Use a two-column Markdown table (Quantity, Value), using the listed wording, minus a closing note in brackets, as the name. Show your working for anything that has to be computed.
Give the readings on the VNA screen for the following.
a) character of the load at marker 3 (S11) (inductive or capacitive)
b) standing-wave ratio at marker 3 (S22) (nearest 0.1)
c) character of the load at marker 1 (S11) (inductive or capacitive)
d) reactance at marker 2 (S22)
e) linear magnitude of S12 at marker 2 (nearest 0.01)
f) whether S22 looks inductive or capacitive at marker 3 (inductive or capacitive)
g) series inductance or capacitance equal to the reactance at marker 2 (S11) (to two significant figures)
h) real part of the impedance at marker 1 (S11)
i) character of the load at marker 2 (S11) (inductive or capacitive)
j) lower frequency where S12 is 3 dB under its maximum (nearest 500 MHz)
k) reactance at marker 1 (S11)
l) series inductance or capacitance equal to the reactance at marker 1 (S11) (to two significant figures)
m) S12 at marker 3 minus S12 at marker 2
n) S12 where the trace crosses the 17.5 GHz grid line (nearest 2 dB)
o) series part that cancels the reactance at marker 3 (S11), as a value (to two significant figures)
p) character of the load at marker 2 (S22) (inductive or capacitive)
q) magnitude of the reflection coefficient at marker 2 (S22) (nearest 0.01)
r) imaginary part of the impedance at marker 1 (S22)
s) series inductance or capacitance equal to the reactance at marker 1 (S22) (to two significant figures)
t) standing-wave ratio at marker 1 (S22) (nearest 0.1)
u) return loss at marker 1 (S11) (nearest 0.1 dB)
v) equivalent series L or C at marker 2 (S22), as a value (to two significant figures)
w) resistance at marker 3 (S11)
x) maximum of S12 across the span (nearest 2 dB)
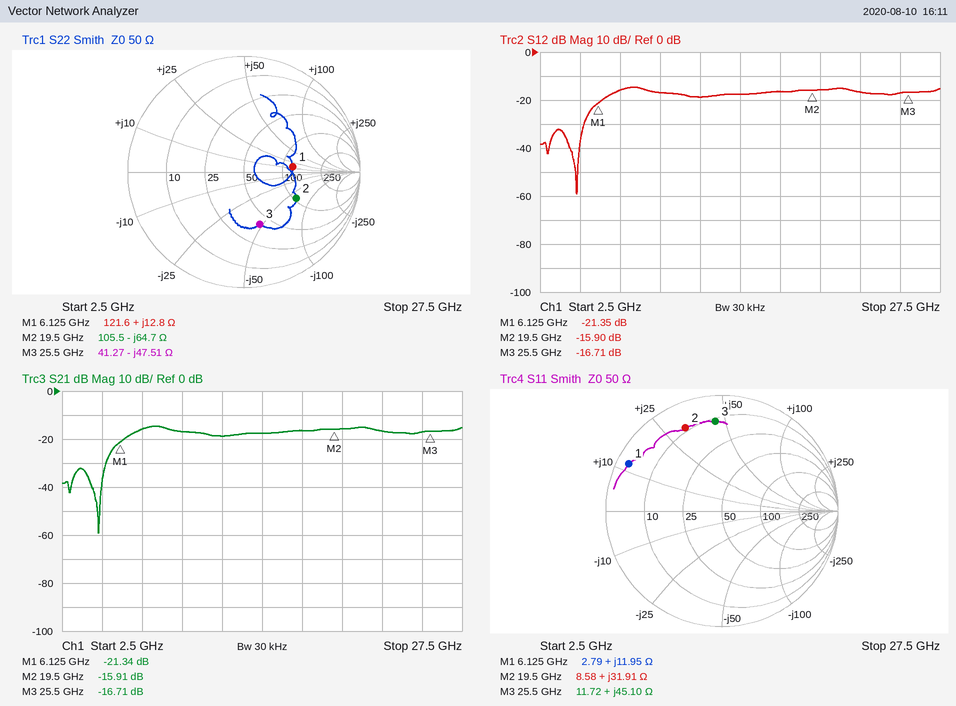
| Quantity | Value |
|---|---|
| character of the load at marker 3 (S11) | inductive |
| standing-wave ratio at marker 3 (S22) | 2.8 |
| character of the load at marker 1 (S11) | inductive |
| reactance at marker 2 | -64.7 Ω |
| linear magnitude of S12 at marker 2 | 10^(-15.9/20) ≈ 0.16 |
| whether S22 looks inductive or capacitive at marker 3 | capacitive |
| series inductance or capacitance equal to the reactance at marker 2 (S11) | L = 31.91 Ω/(2π × 19.5 GHz) ≈ 260 pH |
| real part of the impedance at marker 1 | 2.79 Ω |
| character of the load at marker 2 (S11) | inductive |
| lower frequency where S12 is 3 dB under its maximum | 7.0 GHz |
| reactance at marker 1 | +11.95 Ω |
| series inductance or capacitance equal to the reactance at marker 1 (S11) | L = 11.95 Ω/(2π × 6.125 GHz) ≈ 311 pH, so 310 pH to two significant figures |
| S12 at marker 3 minus S12 at marker 2 | -16.71 − (-15.9) = -0.81 dB |
| S12 where the trace crosses the 17.5 GHz grid line | -16 dB |
| series part that cancels the reactance at marker 3 (S11), as a value | C = 1/(2π × 25.5 GHz × 45.1 Ω) ≈ 138 fF, so 140 fF to two significant figures |
| character of the load at marker 2 (S22) | capacitive |
| magnitude of the reflection coefficient at marker 2 (S22) | 0.51 |
| imaginary part of the impedance at marker 1 | +12.8 Ω |
| series inductance or capacitance equal to the reactance at marker 1 (S22) | L = 12.8 Ω/(2π × 6.125 GHz) ≈ 333 pH, so 330 pH to two significant figures |
| standing-wave ratio at marker 1 (S22) | 2.5 |
| return loss at marker 1 (S11) | 0.9 dB |
| equivalent series L or C at marker 2 (S22), as a value | C = 1/(2π × 19.5 GHz × 64.7 Ω) ≈ 126 fF, so 130 fF to two significant figures |
| resistance at marker 3 | 11.72 Ω |
| maximum of S12 across the span | -14 dB |
